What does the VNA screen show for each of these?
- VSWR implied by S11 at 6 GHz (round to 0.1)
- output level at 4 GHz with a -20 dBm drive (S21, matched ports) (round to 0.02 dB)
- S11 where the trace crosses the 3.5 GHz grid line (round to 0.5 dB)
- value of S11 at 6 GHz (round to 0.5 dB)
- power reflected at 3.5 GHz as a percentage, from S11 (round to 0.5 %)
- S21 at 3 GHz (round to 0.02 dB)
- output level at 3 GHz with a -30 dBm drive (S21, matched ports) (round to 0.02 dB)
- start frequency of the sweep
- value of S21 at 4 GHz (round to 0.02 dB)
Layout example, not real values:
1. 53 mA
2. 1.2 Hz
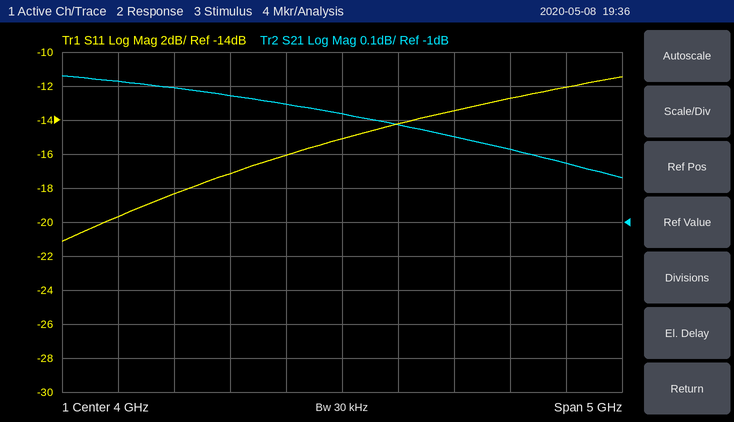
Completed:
1. 1.7
2. -20.68 dBm
3. -16.0 dB
4. -12.0 dB
5. 2.5 %
6. -0.62 dB
7. -30.62 dBm
8. 1.5 GHz
9. -0.68 dB
